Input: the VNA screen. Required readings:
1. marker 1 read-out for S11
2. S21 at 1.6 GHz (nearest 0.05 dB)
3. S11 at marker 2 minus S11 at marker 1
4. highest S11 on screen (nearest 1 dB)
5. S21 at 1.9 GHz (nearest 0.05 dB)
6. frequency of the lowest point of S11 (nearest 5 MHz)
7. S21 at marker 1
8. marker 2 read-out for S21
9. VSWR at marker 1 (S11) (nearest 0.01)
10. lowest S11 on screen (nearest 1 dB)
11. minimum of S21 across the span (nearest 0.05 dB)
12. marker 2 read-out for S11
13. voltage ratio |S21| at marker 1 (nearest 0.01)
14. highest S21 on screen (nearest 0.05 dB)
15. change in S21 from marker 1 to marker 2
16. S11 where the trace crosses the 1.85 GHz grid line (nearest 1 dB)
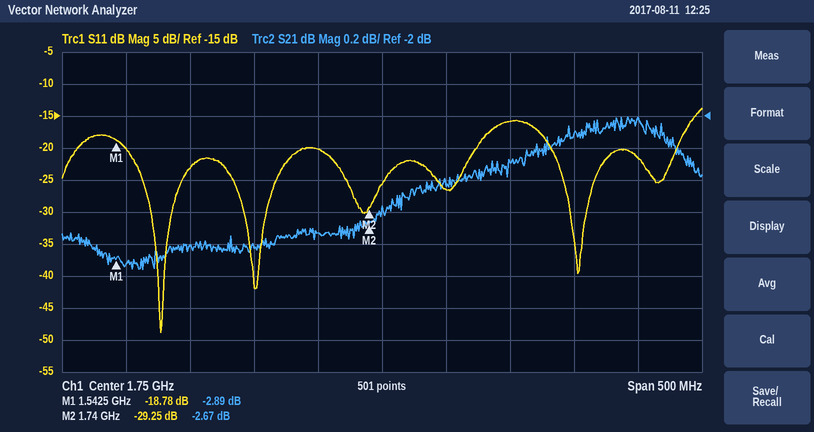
-18.78 dB
-2.80 dB
-10.47 dB
-14 dB
-2.10 dB
1.575 GHz
-2.89 dB
-2.67 dB
1.26
-49 dB
-2.95 dB
-29.25 dB
0.72
-2.00 dB
0.22 dB
-16 dB
